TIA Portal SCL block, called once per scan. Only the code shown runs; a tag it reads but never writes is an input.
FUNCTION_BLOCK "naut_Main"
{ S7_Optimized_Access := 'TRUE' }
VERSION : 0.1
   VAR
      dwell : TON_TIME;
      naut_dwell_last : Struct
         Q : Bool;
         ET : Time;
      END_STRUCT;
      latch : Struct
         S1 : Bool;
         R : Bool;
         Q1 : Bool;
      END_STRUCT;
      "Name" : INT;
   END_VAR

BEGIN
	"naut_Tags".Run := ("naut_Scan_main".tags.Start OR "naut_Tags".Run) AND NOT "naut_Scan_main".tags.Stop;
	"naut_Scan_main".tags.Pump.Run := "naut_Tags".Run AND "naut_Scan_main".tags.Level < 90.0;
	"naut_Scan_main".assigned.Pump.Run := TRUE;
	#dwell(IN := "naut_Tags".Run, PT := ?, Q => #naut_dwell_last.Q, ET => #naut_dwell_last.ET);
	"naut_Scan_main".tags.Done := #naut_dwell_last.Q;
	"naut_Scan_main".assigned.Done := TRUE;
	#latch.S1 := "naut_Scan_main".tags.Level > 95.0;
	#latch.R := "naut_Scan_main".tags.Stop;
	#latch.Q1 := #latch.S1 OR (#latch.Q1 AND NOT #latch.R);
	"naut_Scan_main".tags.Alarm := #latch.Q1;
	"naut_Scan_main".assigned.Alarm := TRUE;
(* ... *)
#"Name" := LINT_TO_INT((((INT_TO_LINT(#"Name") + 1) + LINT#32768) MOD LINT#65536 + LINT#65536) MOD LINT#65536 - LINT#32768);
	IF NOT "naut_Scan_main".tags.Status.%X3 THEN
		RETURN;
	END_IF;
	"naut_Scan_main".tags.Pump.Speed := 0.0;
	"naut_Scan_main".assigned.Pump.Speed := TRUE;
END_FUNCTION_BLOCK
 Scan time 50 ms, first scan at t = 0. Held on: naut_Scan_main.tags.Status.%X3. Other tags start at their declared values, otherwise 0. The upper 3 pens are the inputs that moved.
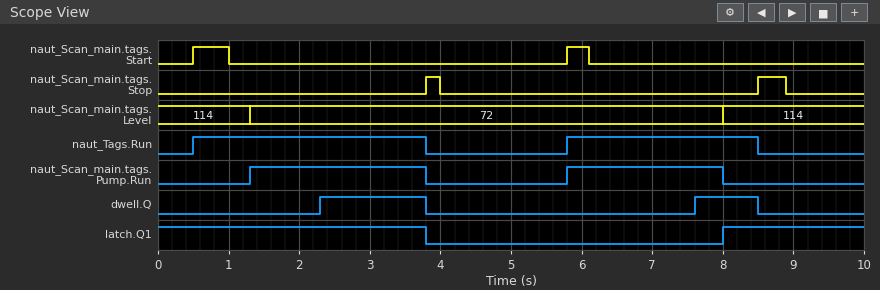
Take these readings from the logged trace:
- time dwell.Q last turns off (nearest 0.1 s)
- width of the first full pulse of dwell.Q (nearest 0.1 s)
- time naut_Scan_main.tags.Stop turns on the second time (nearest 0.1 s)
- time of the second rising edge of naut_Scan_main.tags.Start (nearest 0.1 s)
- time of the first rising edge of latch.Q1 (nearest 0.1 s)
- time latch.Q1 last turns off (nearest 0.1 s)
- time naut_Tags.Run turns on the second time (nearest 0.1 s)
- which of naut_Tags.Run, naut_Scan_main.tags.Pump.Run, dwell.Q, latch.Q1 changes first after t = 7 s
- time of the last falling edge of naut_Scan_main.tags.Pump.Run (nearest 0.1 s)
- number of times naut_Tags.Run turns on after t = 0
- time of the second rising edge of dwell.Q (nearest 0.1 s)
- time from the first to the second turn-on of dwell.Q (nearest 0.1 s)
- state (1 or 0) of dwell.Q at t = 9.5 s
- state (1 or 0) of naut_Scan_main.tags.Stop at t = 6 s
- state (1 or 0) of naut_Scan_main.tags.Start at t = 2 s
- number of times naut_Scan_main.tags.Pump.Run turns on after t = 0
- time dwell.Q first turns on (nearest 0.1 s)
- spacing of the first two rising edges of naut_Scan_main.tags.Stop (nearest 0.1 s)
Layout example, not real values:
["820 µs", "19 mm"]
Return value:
["8.5 s", "1.5 s", "8.5 s", "5.8 s", "8.0 s", "3.8 s", "5.8 s", "dwell.Q", "8.0 s", "2", "7.6 s", "5.3 s", "0", "0", "0", "2", "2.3 s", "4.7 s"]
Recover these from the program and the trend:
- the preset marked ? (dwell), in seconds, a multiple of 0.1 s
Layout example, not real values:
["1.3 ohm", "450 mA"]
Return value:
["1.8 s"]
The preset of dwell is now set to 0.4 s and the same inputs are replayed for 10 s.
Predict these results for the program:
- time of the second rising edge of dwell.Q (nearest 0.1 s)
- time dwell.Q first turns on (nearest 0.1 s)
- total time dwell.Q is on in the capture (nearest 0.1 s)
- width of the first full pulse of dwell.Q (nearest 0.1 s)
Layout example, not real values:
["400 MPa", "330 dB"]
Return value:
["6.2 s", "0.9 s", "5.2 s", "2.9 s"]
